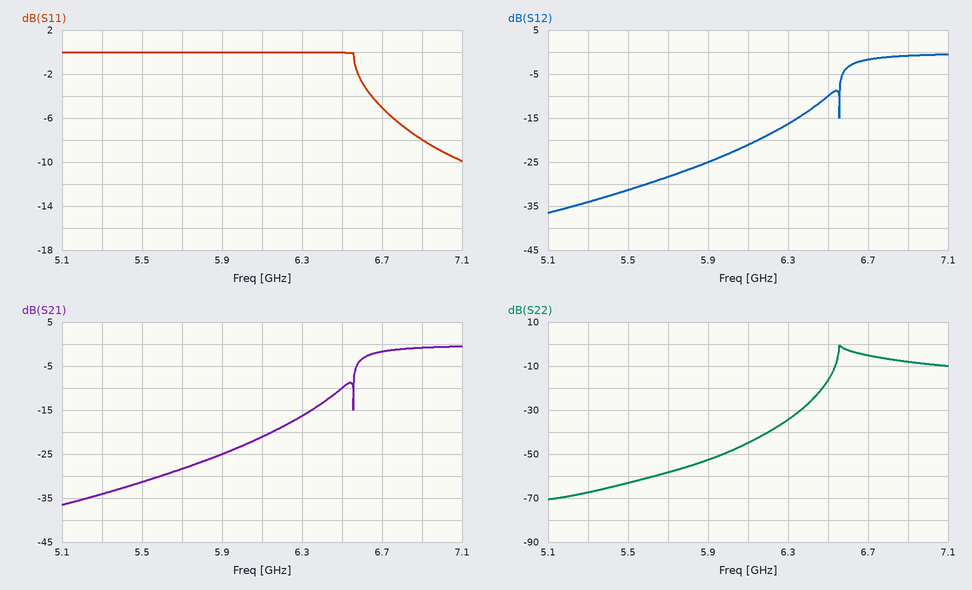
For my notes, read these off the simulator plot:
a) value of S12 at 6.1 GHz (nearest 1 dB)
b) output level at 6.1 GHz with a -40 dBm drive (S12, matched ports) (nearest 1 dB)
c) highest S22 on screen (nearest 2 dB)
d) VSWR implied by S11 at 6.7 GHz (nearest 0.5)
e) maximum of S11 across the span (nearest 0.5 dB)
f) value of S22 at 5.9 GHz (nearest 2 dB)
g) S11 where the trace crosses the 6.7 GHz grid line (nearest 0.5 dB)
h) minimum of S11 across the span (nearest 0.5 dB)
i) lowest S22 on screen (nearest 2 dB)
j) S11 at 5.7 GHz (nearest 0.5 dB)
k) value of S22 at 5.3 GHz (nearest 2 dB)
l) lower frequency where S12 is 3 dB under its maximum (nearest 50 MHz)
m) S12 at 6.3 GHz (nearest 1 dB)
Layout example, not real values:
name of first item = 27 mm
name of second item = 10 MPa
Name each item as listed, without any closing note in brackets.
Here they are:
value of S12 at 6.1 GHz = -21 dB
output level at 6.1 GHz with a -40 dBm drive (S12, matched ports) = -61 dBm
highest S22 on screen = 0 dB
VSWR implied by S11 at 6.7 GHz = 3.5
maximum of S11 across the span = 0.0 dB
value of S22 at 5.9 GHz = -52 dB
S11 where the trace crosses the 6.7 GHz grid line = -5.0 dB
minimum of S11 across the span = -10.0 dB
lowest S22 on screen = -70 dB
S11 at 5.7 GHz = 0.0 dB
value of S22 at 5.3 GHz = -68 dB
lower frequency where S12 is 3 dB under its maximum = 6.60 GHz
S12 at 6.3 GHz = -16 dB
